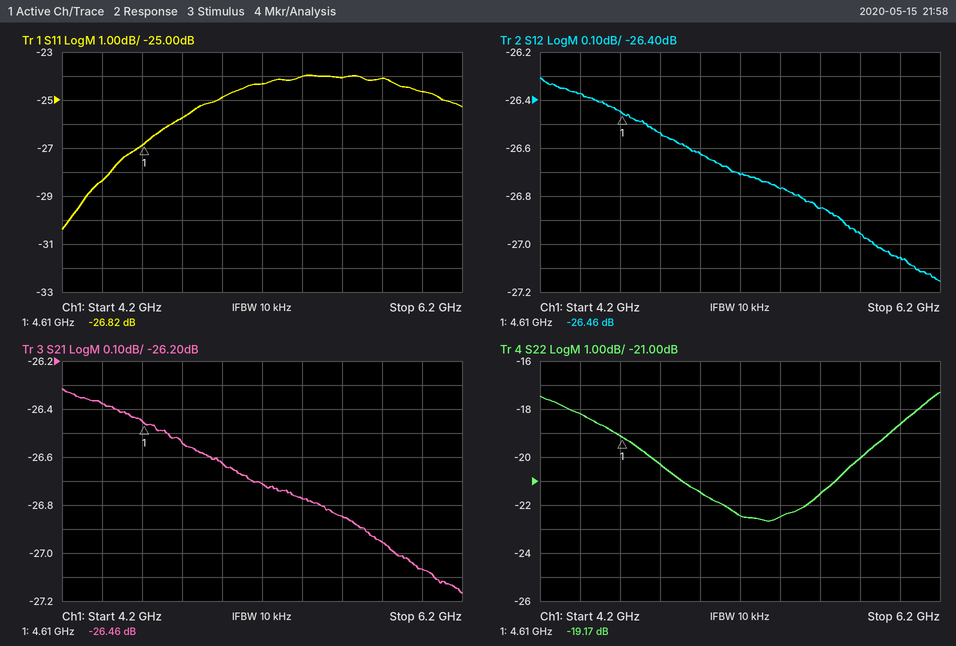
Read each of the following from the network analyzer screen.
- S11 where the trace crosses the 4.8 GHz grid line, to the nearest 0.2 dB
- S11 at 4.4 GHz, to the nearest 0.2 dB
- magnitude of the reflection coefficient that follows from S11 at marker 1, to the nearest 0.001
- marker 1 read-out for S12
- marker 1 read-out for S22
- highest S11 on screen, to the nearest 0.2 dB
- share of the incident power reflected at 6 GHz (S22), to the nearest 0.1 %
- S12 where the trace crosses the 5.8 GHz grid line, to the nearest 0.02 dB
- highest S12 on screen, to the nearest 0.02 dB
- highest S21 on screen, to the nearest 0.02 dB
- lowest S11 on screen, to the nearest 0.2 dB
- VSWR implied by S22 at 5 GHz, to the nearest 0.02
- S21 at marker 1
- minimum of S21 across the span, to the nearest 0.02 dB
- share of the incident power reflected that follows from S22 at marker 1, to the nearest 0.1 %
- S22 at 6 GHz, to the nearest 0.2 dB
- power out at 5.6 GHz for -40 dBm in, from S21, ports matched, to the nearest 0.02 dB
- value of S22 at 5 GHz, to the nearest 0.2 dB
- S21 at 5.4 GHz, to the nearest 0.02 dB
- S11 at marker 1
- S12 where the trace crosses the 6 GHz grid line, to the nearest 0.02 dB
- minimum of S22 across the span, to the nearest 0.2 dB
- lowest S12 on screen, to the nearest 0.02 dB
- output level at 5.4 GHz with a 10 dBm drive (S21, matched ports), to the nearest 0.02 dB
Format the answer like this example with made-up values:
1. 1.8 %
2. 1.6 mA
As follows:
1. -25.8 dB
2. -28.4 dB
3. 0.046
4. -26.46 dB
5. -19.17 dB
6. -24.0 dB
7. 1.4 %
8. -26.96 dB
9. -26.30 dB
10. -26.32 dB
11. -30.4 dB
12. 1.18
13. -26.46 dB
14. -27.16 dB
15. 1.2 %
16. -18.6 dB
17. -66.84 dBm
18. -21.4 dB
19. -26.78 dB
20. -26.82 dB
21. -27.06 dB
22. -22.6 dB
23. -27.16 dB
24. -16.78 dBm
